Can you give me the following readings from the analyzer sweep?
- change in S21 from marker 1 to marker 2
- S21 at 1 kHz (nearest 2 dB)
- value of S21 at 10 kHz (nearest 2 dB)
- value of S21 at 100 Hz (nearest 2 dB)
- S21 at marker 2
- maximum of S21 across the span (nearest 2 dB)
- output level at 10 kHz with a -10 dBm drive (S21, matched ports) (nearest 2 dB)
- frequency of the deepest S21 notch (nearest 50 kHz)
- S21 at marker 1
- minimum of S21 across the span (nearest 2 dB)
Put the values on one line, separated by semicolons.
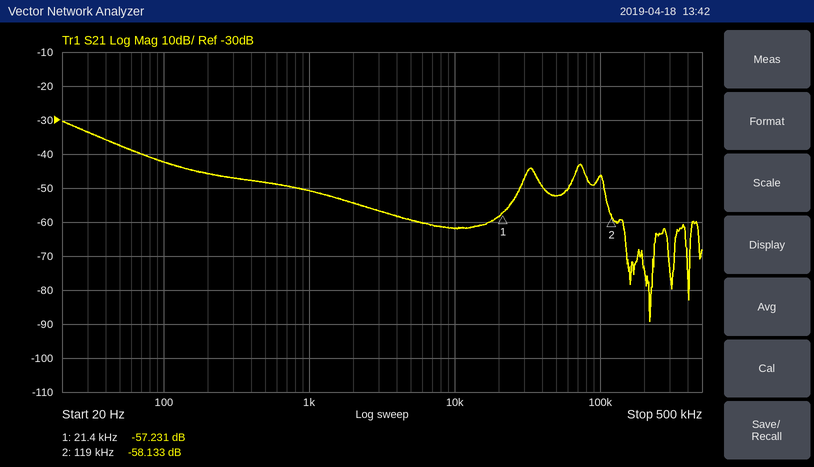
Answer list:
-0.902 dB; -50 dB; -62 dB; -42 dB; -58.133 dB; -30 dB; -72 dBm; 200 kHz; -57.231 dB; -90 dB
